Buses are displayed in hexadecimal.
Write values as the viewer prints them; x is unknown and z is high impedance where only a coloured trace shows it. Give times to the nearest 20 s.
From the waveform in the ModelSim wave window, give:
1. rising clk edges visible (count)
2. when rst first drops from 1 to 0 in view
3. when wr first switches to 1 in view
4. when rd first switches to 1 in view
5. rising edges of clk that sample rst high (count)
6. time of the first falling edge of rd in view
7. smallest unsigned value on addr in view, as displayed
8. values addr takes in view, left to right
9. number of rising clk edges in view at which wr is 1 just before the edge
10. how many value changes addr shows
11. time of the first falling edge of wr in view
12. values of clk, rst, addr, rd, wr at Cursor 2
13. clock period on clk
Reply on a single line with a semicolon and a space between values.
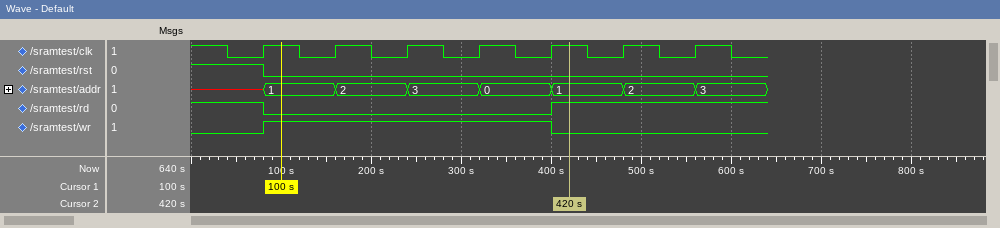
7; 80 s; 80 s; 400 s; 1; 80 s; 0; x, 1, 2, 3, 0, 1, 2, 3; 4; 7; 400 s; clk=1, rst=0, addr=1, rd=1, wr=0; 80 s
